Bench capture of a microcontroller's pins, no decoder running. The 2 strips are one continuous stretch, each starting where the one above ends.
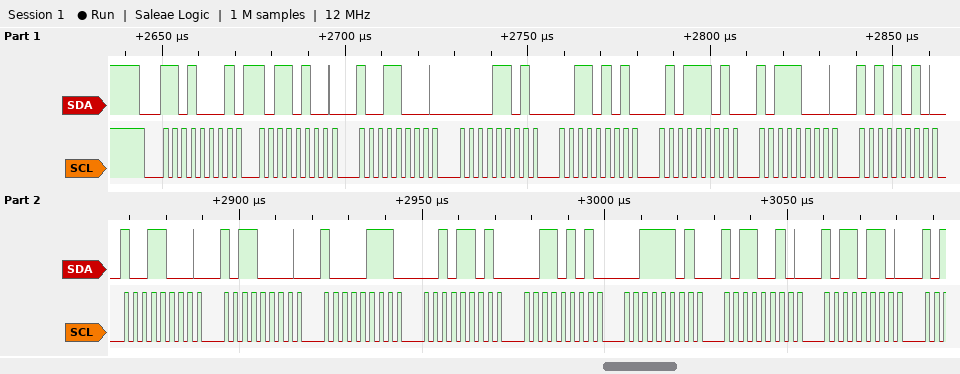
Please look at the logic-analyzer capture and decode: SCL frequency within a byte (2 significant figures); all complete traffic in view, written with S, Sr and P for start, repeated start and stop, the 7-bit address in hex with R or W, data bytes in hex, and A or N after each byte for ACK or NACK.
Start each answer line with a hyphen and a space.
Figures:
- 400 kHz
- S 68R A B4 A 98 A 0D A 35 A 5D A B8 A AA A 98 A B0 A 87 A 2D A 35 A 3D A B2 A B6 A
